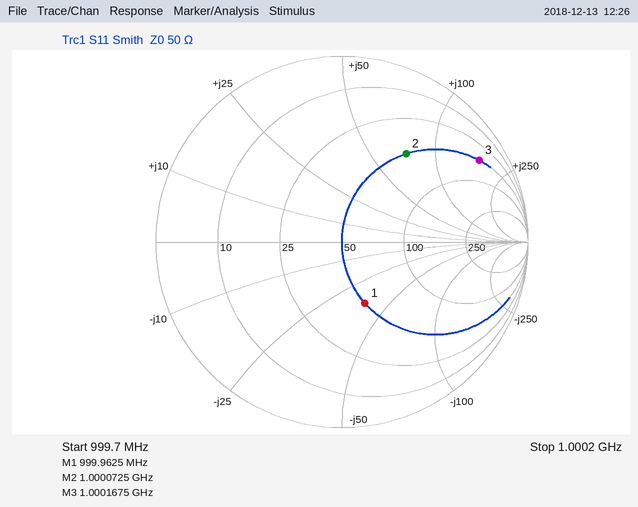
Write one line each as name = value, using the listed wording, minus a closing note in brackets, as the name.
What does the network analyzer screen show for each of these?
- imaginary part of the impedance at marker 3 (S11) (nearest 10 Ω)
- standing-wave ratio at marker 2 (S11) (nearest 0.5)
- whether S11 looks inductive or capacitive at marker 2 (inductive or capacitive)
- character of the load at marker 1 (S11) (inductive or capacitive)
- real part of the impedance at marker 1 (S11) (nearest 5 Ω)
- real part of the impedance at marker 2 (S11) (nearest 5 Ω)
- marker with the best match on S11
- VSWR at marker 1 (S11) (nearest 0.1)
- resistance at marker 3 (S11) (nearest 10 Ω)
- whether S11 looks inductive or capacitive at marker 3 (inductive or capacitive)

imaginary part of the impedance at marker 3 (S11) = +170 Ω
standing-wave ratio at marker 2 (S11) = 4.0
whether S11 looks inductive or capacitive at marker 2 = inductive
character of the load at marker 1 (S11) = capacitive
real part of the impedance at marker 1 (S11) = 50 Ω
real part of the impedance at marker 2 (S11) = 50 Ω
marker with the best match on S11 = marker 1
VSWR at marker 1 (S11) = 2.1
resistance at marker 3 (S11) = 50 Ω
whether S11 looks inductive or capacitive at marker 3 = inductive
